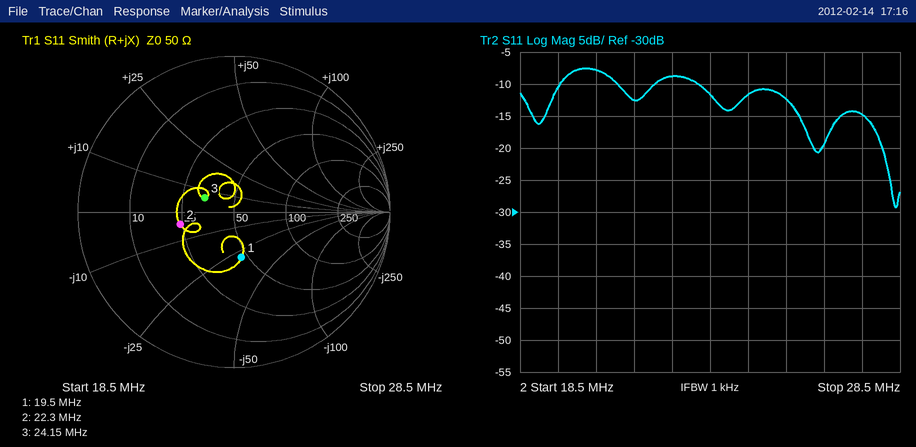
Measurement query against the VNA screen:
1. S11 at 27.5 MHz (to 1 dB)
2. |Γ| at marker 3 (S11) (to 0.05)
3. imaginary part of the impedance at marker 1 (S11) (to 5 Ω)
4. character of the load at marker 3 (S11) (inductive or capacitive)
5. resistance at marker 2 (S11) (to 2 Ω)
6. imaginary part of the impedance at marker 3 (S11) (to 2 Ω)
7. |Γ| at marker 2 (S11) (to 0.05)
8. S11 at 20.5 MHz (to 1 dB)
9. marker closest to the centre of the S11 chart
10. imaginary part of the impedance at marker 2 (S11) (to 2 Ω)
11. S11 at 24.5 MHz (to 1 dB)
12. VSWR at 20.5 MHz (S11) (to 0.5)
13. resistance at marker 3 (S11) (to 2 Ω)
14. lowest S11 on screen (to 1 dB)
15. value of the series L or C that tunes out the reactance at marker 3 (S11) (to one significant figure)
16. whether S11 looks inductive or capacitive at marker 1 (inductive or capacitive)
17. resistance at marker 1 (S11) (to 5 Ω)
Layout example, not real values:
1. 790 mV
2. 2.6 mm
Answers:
1. -15 dB
2. 0.20
3. -30 Ω
4. inductive
5. 24 Ω
6. +6 Ω
7. 0.35
8. -8 dB
9. marker 3
10. -4 Ω
11. -12 dB
12. 2.5
13. 34 Ω
14. -29 dB
15. 1 nF
16. capacitive
17. 45 Ω
